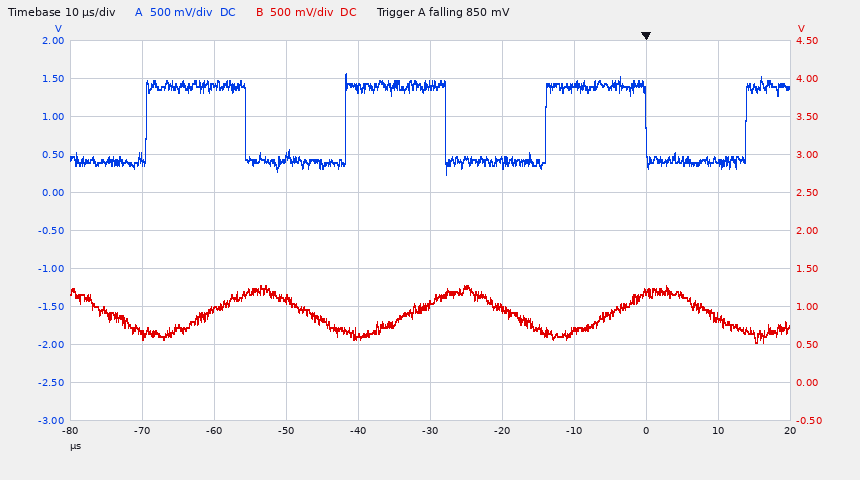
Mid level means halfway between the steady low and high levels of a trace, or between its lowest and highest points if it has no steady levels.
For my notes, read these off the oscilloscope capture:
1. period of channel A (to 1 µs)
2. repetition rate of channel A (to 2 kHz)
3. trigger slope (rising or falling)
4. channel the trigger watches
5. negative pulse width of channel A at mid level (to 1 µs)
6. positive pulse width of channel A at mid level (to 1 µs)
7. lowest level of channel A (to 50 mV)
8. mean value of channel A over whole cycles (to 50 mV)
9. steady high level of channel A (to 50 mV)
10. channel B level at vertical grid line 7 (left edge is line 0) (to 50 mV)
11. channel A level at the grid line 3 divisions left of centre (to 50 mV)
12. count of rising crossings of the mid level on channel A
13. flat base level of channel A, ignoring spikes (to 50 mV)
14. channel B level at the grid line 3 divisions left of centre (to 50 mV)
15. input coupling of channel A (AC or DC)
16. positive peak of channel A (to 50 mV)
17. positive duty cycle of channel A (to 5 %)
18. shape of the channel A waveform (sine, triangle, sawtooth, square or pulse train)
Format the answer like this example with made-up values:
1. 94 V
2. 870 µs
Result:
1. 28 µs
2. 36 kHz
3. falling
4. channel A
5. 14 µs
6. 14 µs
7. 250 mV
8. 900 mV
9. 1.40 V
10. 700 mV
11. 1.40 V
12. 4
13. 400 mV
14. 950 mV
15. DC
16. 1.55 V
17. 50 %
18. square
